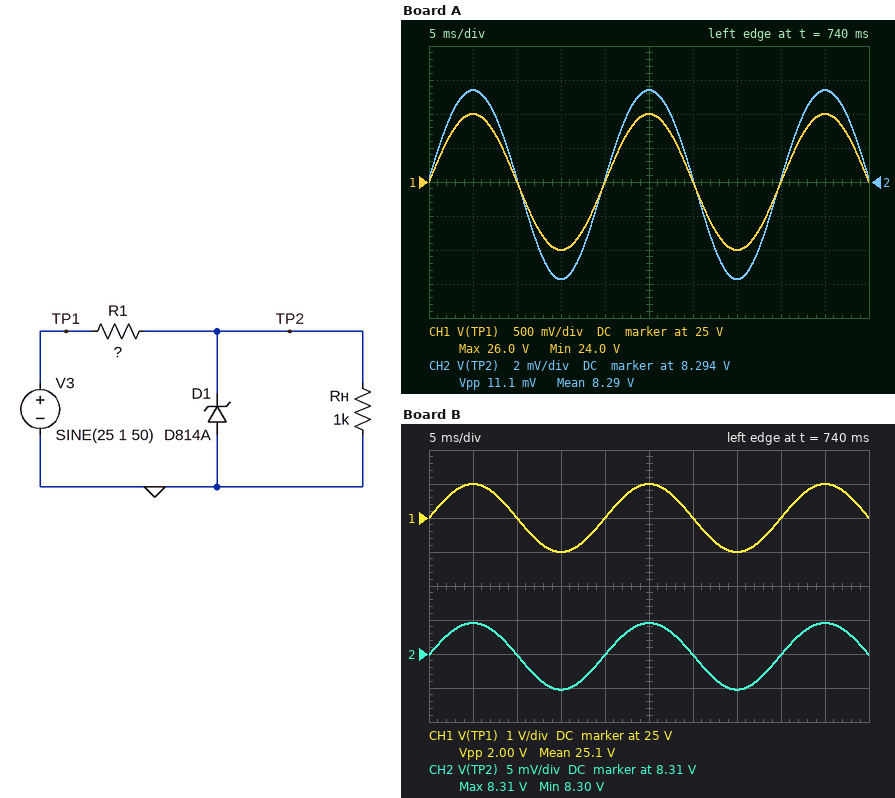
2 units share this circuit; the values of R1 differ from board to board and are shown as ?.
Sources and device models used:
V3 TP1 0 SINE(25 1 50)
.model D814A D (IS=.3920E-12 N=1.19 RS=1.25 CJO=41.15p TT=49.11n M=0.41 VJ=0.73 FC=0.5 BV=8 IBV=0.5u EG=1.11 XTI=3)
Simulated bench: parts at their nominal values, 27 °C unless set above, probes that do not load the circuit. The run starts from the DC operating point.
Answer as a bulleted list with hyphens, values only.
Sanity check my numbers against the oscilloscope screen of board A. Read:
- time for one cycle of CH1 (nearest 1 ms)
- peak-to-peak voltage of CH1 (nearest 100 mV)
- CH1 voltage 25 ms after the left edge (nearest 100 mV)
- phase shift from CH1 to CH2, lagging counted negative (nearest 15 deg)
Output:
- 20 ms
- 2.0 V
- 26.0 V
- 0 deg
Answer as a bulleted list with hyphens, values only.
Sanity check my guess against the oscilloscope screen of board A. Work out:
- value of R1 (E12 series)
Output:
- 1.2 kΩ
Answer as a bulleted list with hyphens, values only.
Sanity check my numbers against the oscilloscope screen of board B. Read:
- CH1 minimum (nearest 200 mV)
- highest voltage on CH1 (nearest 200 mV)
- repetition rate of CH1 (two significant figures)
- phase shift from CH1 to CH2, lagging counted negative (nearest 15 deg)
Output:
- 24.0 V
- 26.0 V
- 50 Hz
- 0 deg
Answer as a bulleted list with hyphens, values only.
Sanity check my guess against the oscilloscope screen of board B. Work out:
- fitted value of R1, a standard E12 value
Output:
- 1 kΩ
